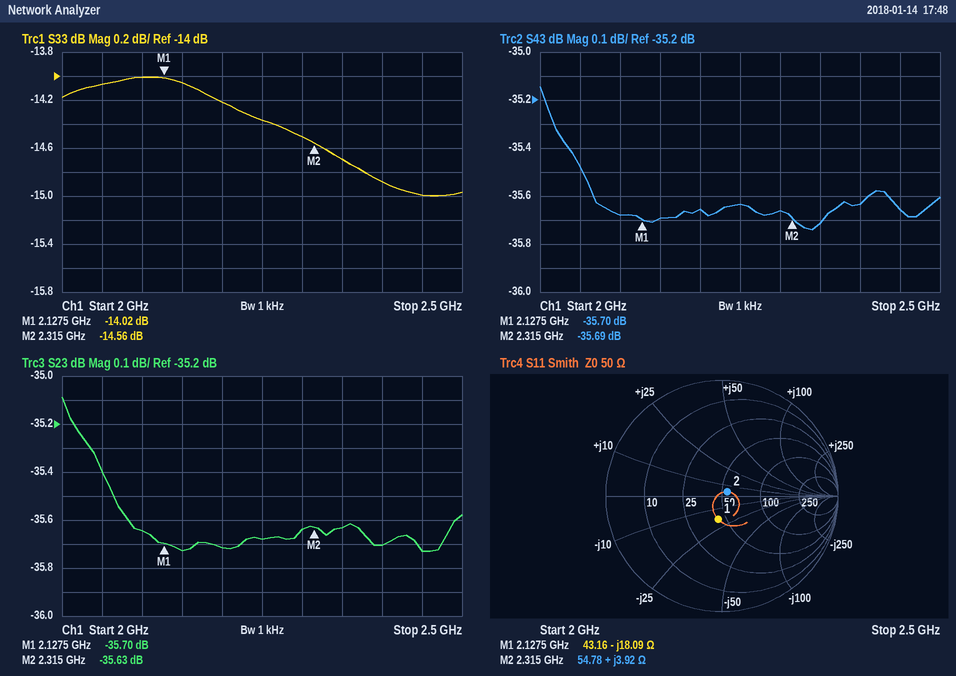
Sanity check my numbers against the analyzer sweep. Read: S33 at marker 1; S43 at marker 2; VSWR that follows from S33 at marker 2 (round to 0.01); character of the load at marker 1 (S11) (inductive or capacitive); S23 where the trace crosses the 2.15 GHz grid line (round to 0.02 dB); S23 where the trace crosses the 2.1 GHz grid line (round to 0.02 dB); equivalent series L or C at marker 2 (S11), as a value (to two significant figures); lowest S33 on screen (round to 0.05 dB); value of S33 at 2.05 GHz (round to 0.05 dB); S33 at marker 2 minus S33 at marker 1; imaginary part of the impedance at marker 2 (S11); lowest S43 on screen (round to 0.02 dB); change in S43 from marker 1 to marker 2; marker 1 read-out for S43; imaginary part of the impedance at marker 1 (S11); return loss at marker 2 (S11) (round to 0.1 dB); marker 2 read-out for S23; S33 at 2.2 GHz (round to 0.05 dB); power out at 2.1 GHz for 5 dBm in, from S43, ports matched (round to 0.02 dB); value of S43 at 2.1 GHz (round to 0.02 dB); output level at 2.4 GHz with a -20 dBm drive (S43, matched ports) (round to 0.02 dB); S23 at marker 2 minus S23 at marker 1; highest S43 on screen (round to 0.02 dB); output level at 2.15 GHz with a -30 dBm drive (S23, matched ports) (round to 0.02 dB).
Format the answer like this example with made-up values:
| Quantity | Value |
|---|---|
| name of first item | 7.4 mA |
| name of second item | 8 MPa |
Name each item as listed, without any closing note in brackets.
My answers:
| Quantity | Value |
|---|---|
| S33 at marker 1 | -14.02 dB |
| S43 at marker 2 | -35.69 dB |
| VSWR that follows from S33 at marker 2 | 1.46 |
| character of the load at marker 1 (S11) | capacitive |
| S23 where the trace crosses the 2.15 GHz grid line | -35.72 dB |
| S23 where the trace crosses the 2.1 GHz grid line | -35.64 dB |
| equivalent series L or C at marker 2 (S11), as a value | 270 pH |
| lowest S33 on screen | -15.00 dB |
| value of S33 at 2.05 GHz | -14.05 dB |
| S33 at marker 2 minus S33 at marker 1 | -0.54 dB |
| imaginary part of the impedance at marker 2 | +3.92 Ω |
| lowest S43 on screen | -35.74 dB |
| change in S43 from marker 1 to marker 2 | 0.01 dB |
| marker 1 read-out for S43 | -35.70 dB |
| imaginary part of the impedance at marker 1 | -18.09 Ω |
| return loss at marker 2 (S11) | 24.6 dB |
| marker 2 read-out for S23 | -35.63 dB |
| S33 at 2.2 GHz | -14.20 dB |
| power out at 2.1 GHz for 5 dBm in, from S43, ports matched | -30.68 dBm |
| value of S43 at 2.1 GHz | -35.68 dB |
| output level at 2.4 GHz with a -20 dBm drive (S43, matched ports) | -55.64 dBm |
| S23 at marker 2 minus S23 at marker 1 | 0.07 dB |
| highest S43 on screen | -35.14 dB |
| output level at 2.15 GHz with a -30 dBm drive (S23, matched ports) | -65.72 dBm |
